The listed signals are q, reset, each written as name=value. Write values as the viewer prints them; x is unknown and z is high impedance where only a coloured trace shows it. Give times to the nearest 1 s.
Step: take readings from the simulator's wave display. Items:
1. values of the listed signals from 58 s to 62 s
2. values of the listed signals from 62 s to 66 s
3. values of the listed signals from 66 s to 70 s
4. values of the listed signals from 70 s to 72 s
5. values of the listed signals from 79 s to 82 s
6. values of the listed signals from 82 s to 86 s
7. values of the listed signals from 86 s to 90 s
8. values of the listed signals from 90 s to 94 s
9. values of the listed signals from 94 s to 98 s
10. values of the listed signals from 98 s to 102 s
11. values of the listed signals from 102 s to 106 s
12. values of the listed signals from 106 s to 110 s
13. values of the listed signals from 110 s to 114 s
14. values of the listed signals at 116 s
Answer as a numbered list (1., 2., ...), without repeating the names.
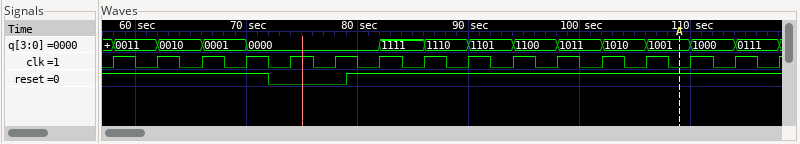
1. q=0011, reset=1
2. q=0010, reset=1
3. q=0001, reset=1
4. q=0000, reset=1
5. q=0000, reset=1
6. q=1111, reset=1
7. q=1110, reset=1
8. q=1101, reset=1
9. q=1100, reset=1
10. q=1011, reset=1
11. q=1010, reset=1
12. q=1001, reset=1
13. q=1000, reset=1
14. q=0111, reset=1
